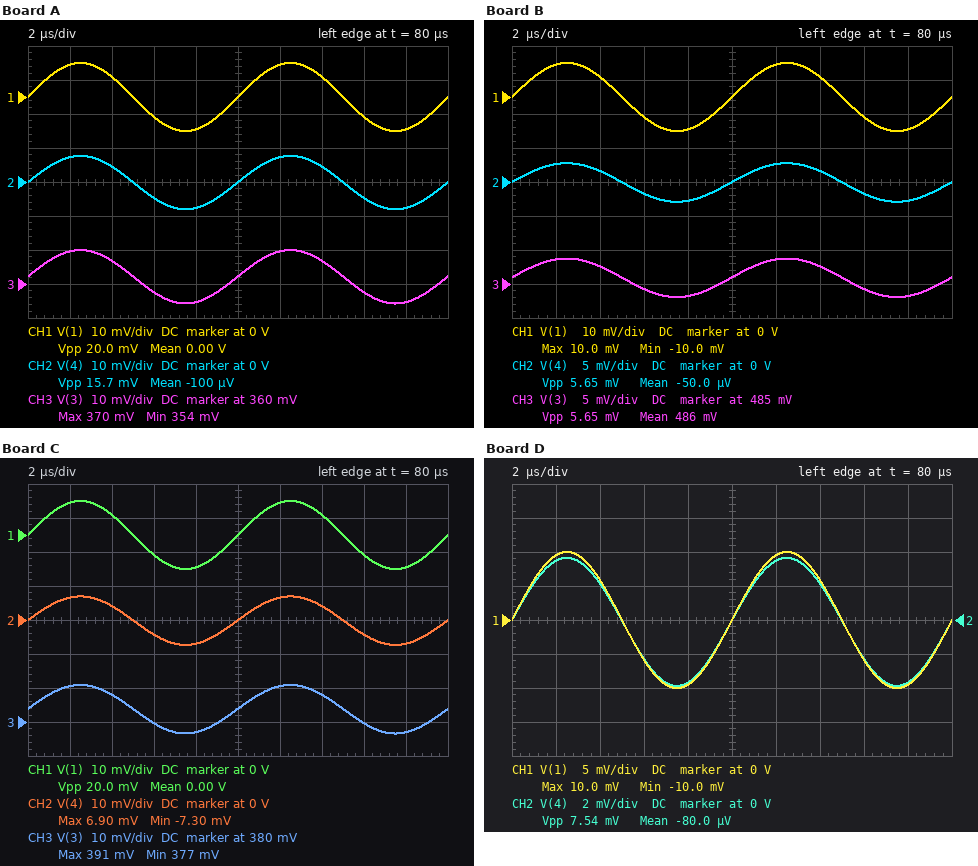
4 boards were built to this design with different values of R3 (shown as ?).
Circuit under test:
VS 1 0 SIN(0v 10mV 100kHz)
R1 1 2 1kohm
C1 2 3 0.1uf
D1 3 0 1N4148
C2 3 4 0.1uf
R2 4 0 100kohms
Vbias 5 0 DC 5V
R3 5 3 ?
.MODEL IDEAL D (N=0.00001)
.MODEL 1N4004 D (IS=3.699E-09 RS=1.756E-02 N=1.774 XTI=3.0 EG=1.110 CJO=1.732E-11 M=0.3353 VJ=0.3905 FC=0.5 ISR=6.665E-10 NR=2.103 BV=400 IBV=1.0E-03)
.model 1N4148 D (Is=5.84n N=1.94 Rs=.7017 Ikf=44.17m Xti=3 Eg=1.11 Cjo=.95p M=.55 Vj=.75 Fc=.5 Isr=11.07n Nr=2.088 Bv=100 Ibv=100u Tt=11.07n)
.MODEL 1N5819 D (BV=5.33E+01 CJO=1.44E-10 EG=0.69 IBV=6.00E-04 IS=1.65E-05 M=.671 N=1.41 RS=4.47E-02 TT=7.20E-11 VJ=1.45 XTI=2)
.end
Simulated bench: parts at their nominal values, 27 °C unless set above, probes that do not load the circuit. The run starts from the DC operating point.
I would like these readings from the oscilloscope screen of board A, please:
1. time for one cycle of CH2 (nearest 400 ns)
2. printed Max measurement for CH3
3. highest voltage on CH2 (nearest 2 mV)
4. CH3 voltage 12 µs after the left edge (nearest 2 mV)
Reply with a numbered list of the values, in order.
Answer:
1. 10.0 µs
2. 370 mV
3. 8 mV
4. 370 mV
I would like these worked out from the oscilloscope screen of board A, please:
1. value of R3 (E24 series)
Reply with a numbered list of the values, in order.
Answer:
1. 330 kΩ
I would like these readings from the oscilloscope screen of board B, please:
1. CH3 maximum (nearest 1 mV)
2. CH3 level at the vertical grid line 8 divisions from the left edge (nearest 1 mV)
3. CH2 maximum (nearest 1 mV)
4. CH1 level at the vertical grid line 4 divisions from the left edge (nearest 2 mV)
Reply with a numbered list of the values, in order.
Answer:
1. 489 mV
2. 484 mV
3. 3 mV
4. -10 mV
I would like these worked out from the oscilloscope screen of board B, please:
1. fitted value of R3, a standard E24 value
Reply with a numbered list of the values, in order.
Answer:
1. 33 kΩ
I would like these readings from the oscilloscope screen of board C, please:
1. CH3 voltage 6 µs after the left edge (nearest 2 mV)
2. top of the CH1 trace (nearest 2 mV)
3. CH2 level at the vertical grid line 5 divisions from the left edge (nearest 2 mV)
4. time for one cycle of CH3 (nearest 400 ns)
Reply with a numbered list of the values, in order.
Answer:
1. 380 mV
2. 10 mV
3. 0 V
4. 10.0 µs
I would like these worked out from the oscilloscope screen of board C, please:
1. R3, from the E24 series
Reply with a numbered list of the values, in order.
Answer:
1. 220 kΩ
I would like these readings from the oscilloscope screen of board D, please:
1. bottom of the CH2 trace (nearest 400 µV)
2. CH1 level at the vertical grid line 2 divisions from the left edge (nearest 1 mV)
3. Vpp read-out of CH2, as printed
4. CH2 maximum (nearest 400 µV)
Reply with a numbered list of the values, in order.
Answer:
1. -4.0 mV
2. 6 mV
3. 7.54 mV
4. 3.6 mV
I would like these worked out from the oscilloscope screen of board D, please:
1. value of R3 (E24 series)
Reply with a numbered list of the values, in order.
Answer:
1. 51 kΩ
